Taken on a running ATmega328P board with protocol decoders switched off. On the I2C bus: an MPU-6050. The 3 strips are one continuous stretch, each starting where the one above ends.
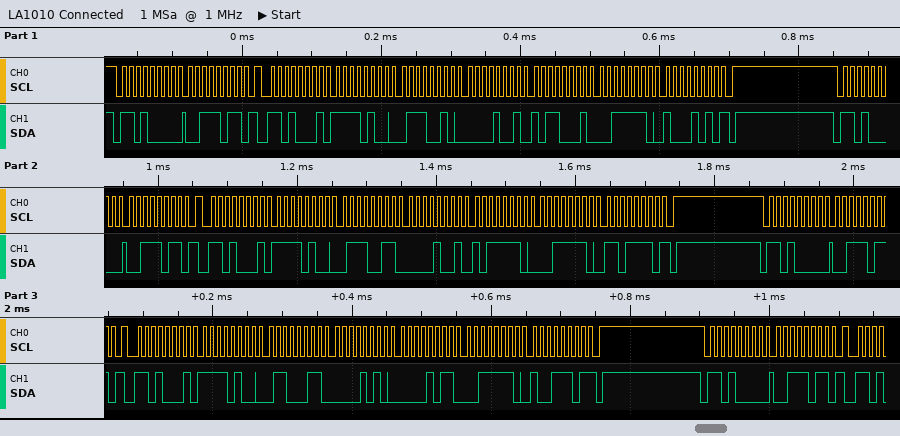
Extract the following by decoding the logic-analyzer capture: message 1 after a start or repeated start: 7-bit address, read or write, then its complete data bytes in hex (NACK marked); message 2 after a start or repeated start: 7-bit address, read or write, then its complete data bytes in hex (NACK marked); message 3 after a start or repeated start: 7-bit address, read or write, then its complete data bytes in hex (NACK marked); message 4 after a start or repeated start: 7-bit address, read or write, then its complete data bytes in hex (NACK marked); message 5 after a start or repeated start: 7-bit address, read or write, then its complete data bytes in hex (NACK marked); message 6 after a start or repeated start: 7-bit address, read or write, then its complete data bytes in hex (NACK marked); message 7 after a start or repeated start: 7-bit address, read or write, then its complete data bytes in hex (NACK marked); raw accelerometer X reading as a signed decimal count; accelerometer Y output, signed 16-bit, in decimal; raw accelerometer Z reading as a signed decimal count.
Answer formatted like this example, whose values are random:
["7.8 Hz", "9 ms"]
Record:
["0x68 write: 3B", "0x68 read: F4 72 09 B1 3E 8A NACK", "0x68 write: 3B", "0x68 read: F4 73 09 BE 3E DE NACK", "0x68 write: 3B", "0x68 read: F4 63 0A 0B 3E 9D NACK", "0x68 write: 3B", "-2958", "2481", "16010"]
